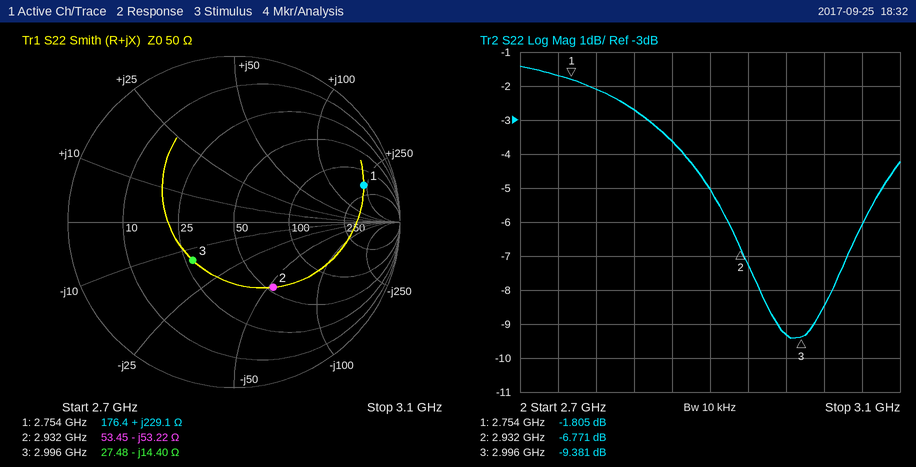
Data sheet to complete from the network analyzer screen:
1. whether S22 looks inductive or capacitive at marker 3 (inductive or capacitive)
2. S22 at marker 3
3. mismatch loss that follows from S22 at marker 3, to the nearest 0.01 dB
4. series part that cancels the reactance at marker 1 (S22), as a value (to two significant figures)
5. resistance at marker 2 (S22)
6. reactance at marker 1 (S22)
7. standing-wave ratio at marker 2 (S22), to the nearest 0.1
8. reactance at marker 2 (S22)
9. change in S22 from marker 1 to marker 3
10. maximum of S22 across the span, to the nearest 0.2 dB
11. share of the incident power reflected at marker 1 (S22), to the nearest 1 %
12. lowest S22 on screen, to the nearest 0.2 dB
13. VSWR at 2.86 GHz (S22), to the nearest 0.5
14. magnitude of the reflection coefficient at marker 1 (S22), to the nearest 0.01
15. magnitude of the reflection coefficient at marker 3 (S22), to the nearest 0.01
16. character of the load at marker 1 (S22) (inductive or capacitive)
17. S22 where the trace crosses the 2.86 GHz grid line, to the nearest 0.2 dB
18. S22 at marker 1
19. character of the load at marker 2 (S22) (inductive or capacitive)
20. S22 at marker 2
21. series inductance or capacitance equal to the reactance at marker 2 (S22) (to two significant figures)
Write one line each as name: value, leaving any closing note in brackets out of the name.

whether S22 looks inductive or capacitive at marker 3: capacitive
S22 at marker 3: -9.381 dB
mismatch loss that follows from S22 at marker 3, to the nearest 0.01 dB: 0.53 dB
series part that cancels the reactance at marker 1 (S22), as a value: 250 fF
resistance at marker 2: 53.45 Ω
reactance at marker 1: +229.1 Ω
standing-wave ratio at marker 2 (S22), to the nearest 0.1: 2.7
reactance at marker 2: -53.22 Ω
change in S22 from marker 1 to marker 3: -7.576 dB
maximum of S22 across the span, to the nearest 0.2 dB: -1.4 dB
share of the incident power reflected at marker 1 (S22), to the nearest 1 %: 66 %
lowest S22 on screen, to the nearest 0.2 dB: -9.4 dB
VSWR at 2.86 GHz (S22), to the nearest 0.5: 5.0
magnitude of the reflection coefficient at marker 1 (S22), to the nearest 0.01: 0.81
magnitude of the reflection coefficient at marker 3 (S22), to the nearest 0.01: 0.34
character of the load at marker 1 (S22): inductive
S22 where the trace crosses the 2.86 GHz grid line, to the nearest 0.2 dB: -3.6 dB
S22 at marker 1: -1.805 dB
character of the load at marker 2 (S22): capacitive
S22 at marker 2: -6.771 dB
series inductance or capacitance equal to the reactance at marker 2 (S22): 1.0 pF
